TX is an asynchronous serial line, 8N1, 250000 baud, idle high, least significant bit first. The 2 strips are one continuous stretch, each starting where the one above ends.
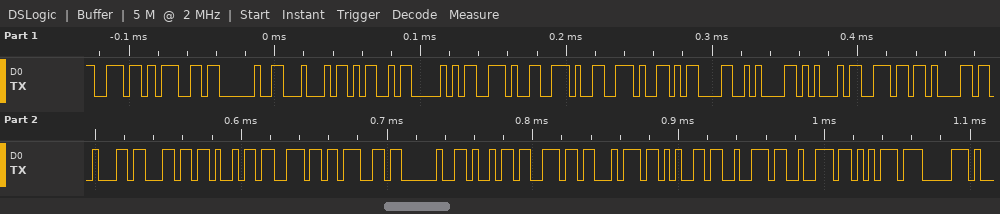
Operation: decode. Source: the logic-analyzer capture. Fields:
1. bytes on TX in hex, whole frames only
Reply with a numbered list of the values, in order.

1. 6E 67 20 44 4D 50 2E 2E 2E 0D 0A 45 6E 61 62 6C 69 6E 67 20 69 6E 74 65 72 72 75 70
